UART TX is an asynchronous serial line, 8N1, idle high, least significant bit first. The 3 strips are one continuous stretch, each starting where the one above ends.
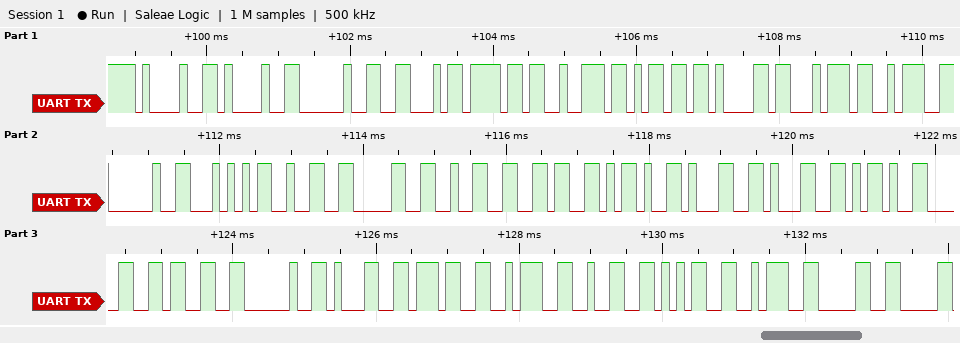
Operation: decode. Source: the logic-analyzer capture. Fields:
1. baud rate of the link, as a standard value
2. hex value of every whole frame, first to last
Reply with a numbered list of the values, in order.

1. 9600 baud
2. 21 21 20 46 6F 72 6D 61 74 3A 20 54 32 30 32 36 2D 31 31 2D 30 33 20 31 37 3A 32 35 3A 30
